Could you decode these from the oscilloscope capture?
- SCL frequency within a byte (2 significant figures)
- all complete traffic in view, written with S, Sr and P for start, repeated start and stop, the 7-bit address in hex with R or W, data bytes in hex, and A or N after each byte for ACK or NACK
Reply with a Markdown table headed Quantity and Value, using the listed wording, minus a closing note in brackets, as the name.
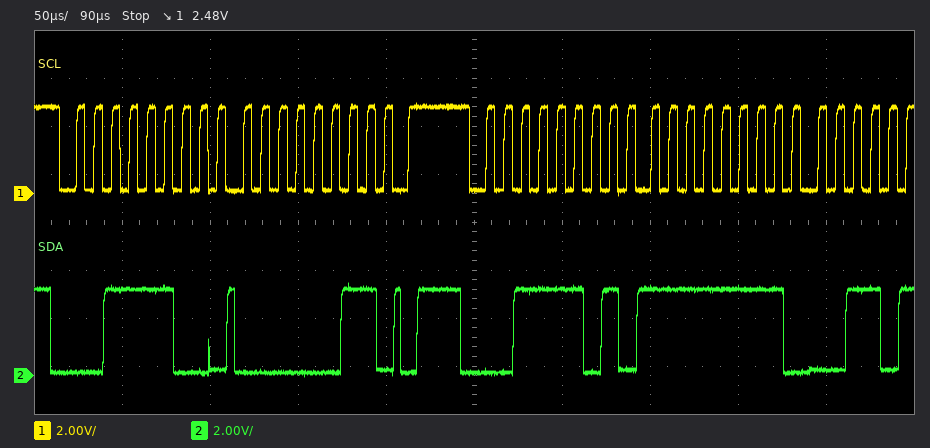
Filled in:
| Quantity | Value |
|---|---|
| SCL frequency within a byte | 100 kHz |
| all complete traffic in view, written with S, Sr and P for start, repeated start and stop, the 7-bit address in hex with R or W, data bytes in hex, and A or N after each byte for ACK or NACK | S 1EW A 03 A P S 1ER A FF A |
